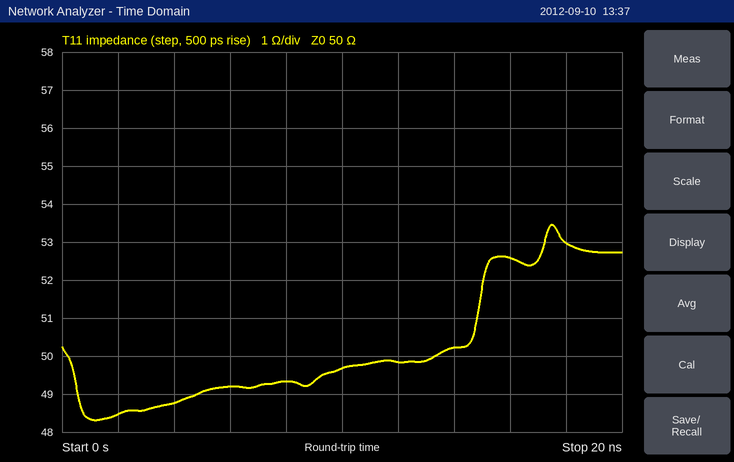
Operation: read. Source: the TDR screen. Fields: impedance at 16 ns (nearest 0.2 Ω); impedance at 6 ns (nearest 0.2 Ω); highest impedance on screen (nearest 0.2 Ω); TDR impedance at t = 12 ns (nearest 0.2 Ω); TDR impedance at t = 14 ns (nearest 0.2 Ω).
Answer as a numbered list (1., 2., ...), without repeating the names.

1. 52.6 Ω
2. 49.2 Ω
3. 53.4 Ω
4. 49.8 Ω
5. 50.2 Ω
